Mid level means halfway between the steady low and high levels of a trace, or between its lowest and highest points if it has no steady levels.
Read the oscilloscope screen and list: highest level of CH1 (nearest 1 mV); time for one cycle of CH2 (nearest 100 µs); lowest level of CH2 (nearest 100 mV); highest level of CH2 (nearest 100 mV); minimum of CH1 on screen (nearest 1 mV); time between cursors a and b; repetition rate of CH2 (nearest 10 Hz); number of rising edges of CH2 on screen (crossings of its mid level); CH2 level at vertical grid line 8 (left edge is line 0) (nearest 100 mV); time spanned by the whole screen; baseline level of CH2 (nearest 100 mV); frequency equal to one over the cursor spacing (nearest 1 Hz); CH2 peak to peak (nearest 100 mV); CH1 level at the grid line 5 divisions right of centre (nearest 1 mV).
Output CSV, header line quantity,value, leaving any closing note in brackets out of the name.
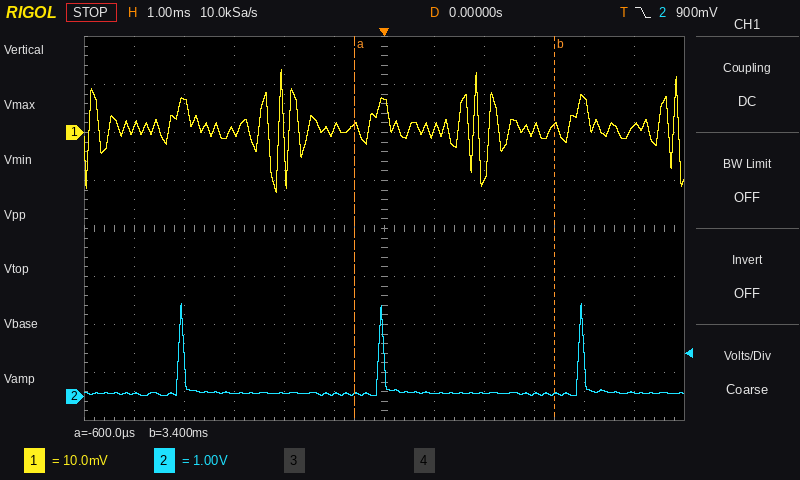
quantity,value
highest level of CH1,13 mV
time for one cycle of CH2,4.0 ms
lowest level of CH2,0.0 V
highest level of CH2,1.9 V
minimum of CH1 on screen,-12 mV
time between cursors a and b,4.0 ms
repetition rate of CH2,250 Hz
number of rising edges of CH2 on screen,3
CH2 level at vertical grid line 8 (left edge is line 0),100 mV
time spanned by the whole screen,12 ms
baseline level of CH2,100 mV
frequency equal to one over the cursor spacing,250 Hz
CH2 peak to peak,1.9 V
CH1 level at the grid line 5 divisions right of centre,1 mV
